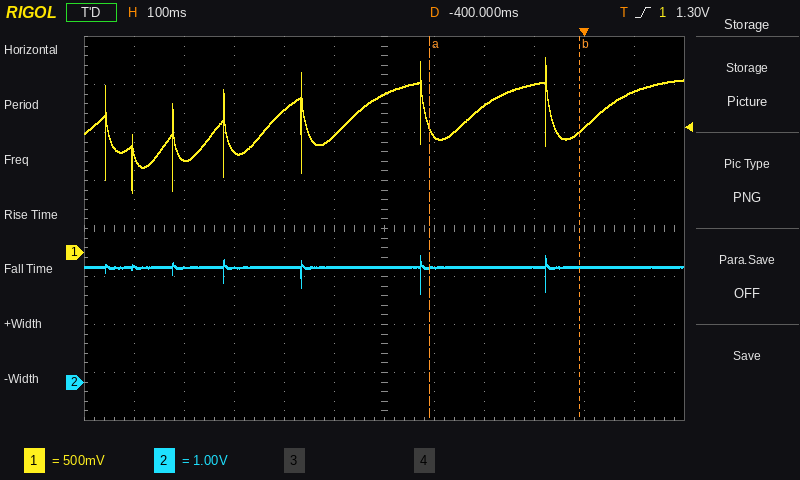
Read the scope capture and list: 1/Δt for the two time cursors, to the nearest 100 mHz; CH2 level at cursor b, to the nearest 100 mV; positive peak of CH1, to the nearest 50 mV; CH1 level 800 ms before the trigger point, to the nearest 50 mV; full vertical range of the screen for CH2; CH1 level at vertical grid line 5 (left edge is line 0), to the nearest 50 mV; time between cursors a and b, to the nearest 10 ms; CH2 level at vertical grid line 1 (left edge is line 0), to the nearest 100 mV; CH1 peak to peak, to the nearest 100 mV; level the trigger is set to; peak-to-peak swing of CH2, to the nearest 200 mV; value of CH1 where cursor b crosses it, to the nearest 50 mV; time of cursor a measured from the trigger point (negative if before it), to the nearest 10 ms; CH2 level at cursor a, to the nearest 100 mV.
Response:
3.3 Hz
2.4 V
2.05 V
950 mV
8 V
1.20 V
300 ms
2.4 V
1.40 V
1.30 V
800 mV
1.25 V
-310 ms
2.4 V
